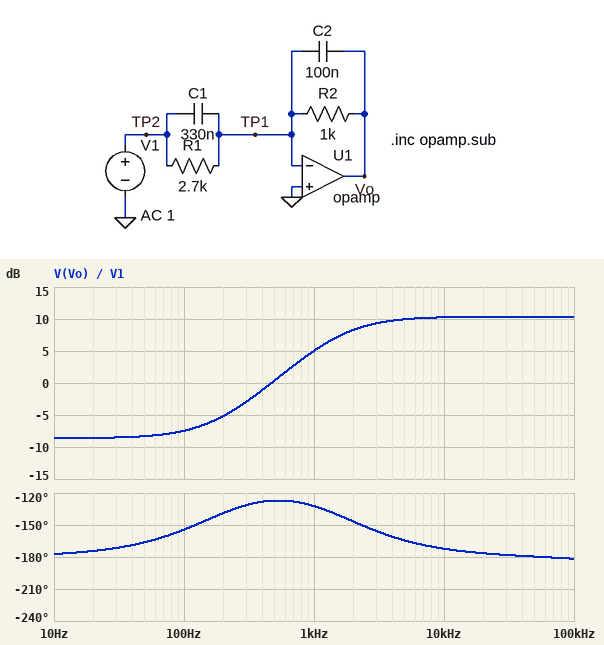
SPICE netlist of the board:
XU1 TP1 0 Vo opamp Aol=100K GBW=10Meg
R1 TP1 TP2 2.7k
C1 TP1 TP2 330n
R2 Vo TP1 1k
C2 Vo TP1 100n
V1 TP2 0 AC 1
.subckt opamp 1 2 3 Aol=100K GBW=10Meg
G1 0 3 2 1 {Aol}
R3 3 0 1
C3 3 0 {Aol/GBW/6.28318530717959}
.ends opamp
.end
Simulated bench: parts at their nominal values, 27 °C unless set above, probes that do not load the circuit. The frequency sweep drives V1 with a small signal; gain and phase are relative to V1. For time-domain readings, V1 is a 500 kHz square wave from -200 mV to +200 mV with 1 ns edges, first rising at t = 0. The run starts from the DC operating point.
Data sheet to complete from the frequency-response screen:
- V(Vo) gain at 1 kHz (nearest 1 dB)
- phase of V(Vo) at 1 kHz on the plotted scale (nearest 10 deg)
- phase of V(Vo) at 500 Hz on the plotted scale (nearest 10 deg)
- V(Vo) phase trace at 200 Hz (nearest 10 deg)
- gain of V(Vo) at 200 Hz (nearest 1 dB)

5 dB
-130 deg
-130 deg
-140 deg
-5 dB
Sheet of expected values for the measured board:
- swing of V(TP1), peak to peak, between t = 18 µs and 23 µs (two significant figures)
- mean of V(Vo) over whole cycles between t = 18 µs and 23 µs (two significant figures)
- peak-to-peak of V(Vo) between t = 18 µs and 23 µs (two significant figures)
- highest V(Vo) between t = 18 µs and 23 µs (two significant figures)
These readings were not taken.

610 mV
-480 mV
1.3 V
190 mV
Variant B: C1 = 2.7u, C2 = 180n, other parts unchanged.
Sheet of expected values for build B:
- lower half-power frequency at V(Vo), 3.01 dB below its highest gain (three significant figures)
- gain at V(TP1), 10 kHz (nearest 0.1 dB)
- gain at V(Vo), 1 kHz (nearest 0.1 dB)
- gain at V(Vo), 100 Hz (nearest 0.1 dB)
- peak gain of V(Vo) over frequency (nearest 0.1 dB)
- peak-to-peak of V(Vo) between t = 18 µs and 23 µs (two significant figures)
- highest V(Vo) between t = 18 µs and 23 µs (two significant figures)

882 Hz
-36.5 dB
21.0 dB
4.7 dB
23.5 dB
5.8 V
290 mV
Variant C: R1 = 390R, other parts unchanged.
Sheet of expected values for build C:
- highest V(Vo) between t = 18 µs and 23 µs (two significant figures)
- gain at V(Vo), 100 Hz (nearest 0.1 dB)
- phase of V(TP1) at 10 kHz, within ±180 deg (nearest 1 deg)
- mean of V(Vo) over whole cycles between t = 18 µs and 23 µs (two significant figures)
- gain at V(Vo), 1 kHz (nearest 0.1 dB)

540 mV
8.2 dB
91 deg
-120 mV
8.9 dB
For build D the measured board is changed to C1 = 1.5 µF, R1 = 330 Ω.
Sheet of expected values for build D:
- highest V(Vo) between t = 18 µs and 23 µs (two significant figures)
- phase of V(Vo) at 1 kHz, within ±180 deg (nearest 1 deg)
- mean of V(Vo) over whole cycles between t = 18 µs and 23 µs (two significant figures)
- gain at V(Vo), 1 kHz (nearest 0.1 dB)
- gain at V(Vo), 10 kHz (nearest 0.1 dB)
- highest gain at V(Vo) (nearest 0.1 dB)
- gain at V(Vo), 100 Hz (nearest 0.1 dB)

960 mV
-140 deg
-2.0 V
18.5 dB
23.4 dB
23.5 dB
10.0 dB
